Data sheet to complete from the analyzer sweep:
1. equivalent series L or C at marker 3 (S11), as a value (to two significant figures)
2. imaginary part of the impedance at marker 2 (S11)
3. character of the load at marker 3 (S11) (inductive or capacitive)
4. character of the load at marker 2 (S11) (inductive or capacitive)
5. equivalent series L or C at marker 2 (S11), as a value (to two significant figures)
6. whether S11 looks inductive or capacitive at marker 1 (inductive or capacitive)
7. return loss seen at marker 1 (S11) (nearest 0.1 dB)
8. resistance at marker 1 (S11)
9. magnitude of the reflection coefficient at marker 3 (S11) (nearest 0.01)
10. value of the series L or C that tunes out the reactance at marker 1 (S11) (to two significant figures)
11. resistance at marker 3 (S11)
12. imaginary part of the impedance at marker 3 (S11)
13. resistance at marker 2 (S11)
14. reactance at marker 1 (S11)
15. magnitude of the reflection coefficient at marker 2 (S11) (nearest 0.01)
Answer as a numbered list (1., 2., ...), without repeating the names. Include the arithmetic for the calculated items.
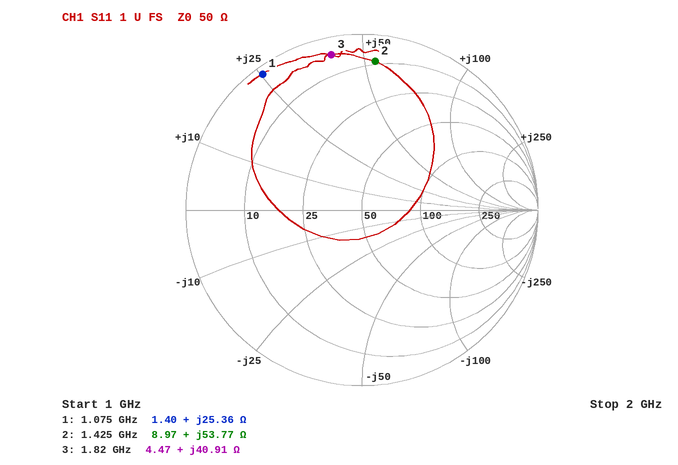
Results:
1. L = 40.91 Ω/(2π × 1.82 GHz) ≈ 3.6 nH
2. +53.77 Ω
3. inductive
4. inductive
5. L = 53.77 Ω/(2π × 1.425 GHz) ≈ 6.0 nH
6. inductive
7. 0.4 dB
8. 1.40 Ω
9. 0.90
10. C = 1/(2π × 1.075 GHz × 25.36 Ω) ≈ 5.8 pF
11. 4.47 Ω
12. +40.91 Ω
13. 8.97 Ω
14. +25.36 Ω
15. 0.85
